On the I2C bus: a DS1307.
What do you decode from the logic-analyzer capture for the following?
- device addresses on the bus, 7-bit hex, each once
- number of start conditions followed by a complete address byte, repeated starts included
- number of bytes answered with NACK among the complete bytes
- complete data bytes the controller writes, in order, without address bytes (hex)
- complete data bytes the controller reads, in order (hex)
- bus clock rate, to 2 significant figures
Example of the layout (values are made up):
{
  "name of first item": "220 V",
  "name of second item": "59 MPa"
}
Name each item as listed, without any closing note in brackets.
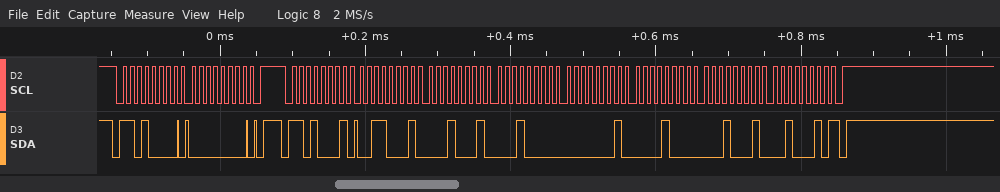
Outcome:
{
  "device addresses on the bus, 7-bit hex, each once": "0x68",
  "number of start conditions followed by a complete address byte, repeated starts included": "2",
  "number of bytes answered with NACK among the complete bytes": "1",
  "complete data bytes the controller writes, in order, without address bytes": "00",
  "complete data bytes the controller reads, in order": "31 11 10 01 08 11 22",
  "bus clock rate, to 2 significant figures": "100 kHz"
}
